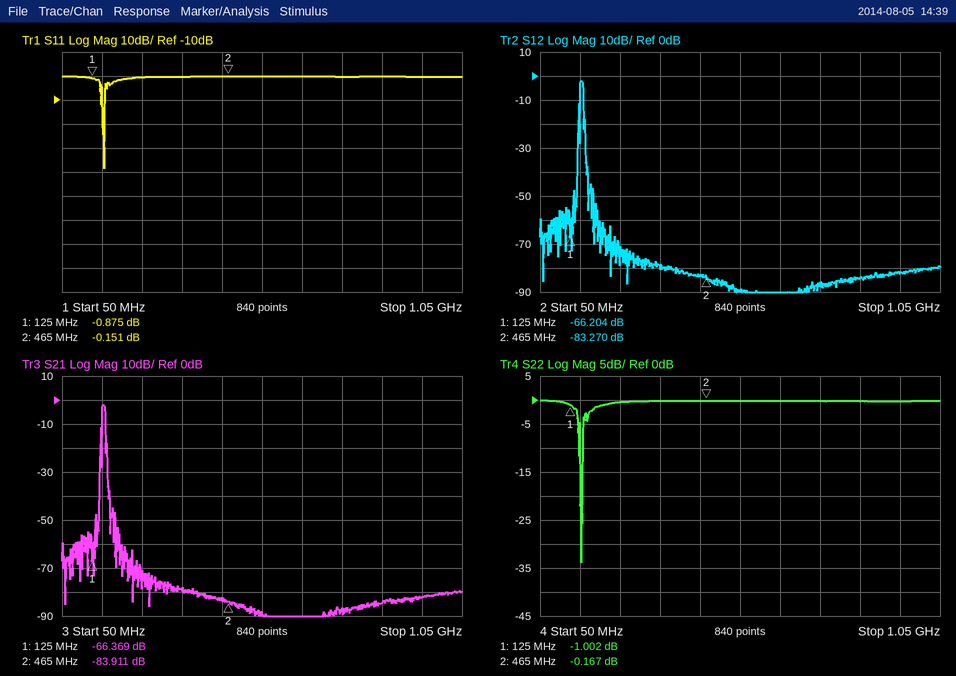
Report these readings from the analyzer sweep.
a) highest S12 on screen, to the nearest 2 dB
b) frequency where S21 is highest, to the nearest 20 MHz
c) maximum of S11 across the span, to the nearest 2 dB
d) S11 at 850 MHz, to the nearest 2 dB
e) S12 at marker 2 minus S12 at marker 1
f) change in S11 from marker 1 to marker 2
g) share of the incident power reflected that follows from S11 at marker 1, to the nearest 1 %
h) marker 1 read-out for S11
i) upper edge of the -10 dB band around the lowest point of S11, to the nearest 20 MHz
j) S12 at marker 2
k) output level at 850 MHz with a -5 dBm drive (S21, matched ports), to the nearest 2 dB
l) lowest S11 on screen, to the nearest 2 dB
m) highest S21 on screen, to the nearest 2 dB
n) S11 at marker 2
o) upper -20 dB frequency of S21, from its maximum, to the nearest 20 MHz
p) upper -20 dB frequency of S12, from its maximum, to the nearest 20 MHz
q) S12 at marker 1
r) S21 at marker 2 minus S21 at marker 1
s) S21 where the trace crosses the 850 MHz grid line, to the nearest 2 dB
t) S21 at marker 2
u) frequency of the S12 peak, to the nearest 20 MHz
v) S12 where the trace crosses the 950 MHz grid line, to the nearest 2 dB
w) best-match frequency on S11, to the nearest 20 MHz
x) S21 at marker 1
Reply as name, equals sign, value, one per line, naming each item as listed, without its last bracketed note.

highest S12 on screen, to the nearest 2 dB = -2 dB
frequency where S21 is highest, to the nearest 20 MHz = 160 MHz
maximum of S11 across the span, to the nearest 2 dB = 0 dB
S11 at 850 MHz, to the nearest 2 dB = 0 dB
S12 at marker 2 minus S12 at marker 1 = -17.066 dB
change in S11 from marker 1 to marker 2 = 0.724 dB
share of the incident power reflected that follows from S11 at marker 1, to the nearest 1 % = 82 %
marker 1 read-out for S11 = -0.875 dB
upper edge of the -10 dB band around the lowest point of S11, to the nearest 20 MHz = 160 MHz
S12 at marker 2 = -83.270 dB
output level at 850 MHz with a -5 dBm drive (S21, matched ports), to the nearest 2 dB = -90 dBm
lowest S11 on screen, to the nearest 2 dB = -38 dB
highest S21 on screen, to the nearest 2 dB = -2 dB
S11 at marker 2 = -0.151 dB
upper -20 dB frequency of S21, from its maximum, to the nearest 20 MHz = 160 MHz
upper -20 dB frequency of S12, from its maximum, to the nearest 20 MHz = 160 MHz
S12 at marker 1 = -66.204 dB
S21 at marker 2 minus S21 at marker 1 = -17.542 dB
S21 where the trace crosses the 850 MHz grid line, to the nearest 2 dB = -84 dB
S21 at marker 2 = -83.911 dB
frequency of the S12 peak, to the nearest 20 MHz = 160 MHz
S12 where the trace crosses the 950 MHz grid line, to the nearest 2 dB = -82 dB
best-match frequency on S11, to the nearest 20 MHz = 160 MHz
S21 at marker 1 = -66.369 dB
